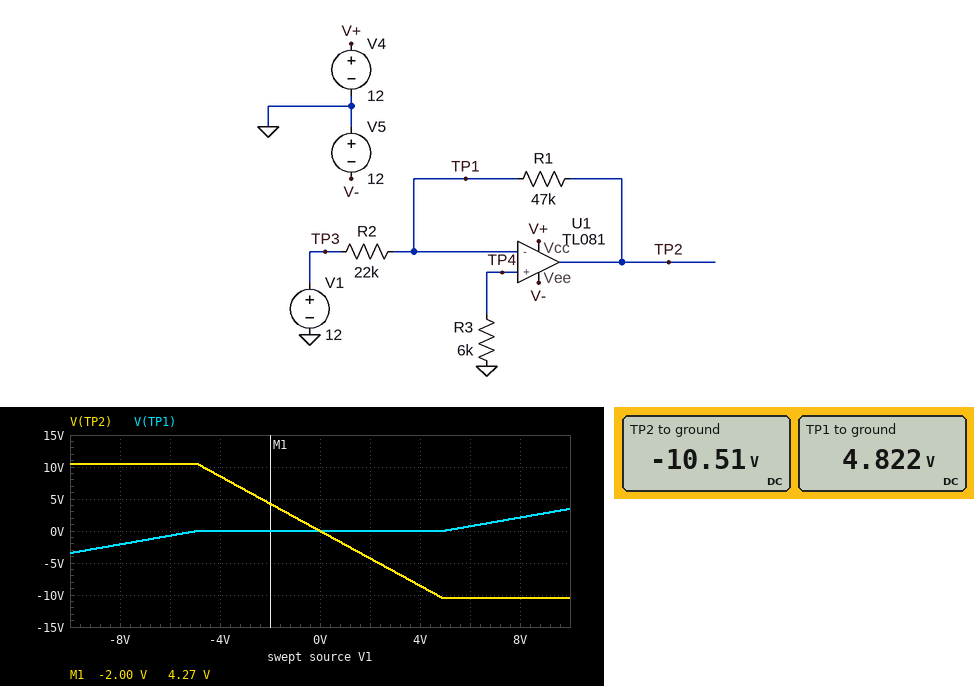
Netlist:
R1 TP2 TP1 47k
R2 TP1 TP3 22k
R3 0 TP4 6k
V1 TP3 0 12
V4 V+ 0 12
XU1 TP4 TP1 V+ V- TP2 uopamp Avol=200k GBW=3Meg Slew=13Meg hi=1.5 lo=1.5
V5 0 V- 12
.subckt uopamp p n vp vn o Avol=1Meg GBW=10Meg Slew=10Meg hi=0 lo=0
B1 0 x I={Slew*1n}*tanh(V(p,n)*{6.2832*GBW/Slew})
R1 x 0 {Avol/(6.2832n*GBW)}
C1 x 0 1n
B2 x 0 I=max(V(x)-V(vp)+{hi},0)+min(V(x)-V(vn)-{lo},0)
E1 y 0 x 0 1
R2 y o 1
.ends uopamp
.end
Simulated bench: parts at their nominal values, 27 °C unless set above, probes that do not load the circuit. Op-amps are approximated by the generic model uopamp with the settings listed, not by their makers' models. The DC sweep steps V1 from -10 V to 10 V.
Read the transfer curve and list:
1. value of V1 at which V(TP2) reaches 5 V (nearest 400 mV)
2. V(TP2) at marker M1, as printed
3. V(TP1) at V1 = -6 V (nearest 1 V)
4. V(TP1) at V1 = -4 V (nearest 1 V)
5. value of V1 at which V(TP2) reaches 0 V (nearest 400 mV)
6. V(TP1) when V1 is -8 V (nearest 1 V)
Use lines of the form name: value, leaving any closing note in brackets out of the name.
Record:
value of V1 at which V(TP2) reaches 5 V: -2.4 V
V(TP2) at marker M1, as printed: 4.27 V
V(TP1) at V1 = -6 V: -1 V
V(TP1) at V1 = -4 V: 0 V
value of V1 at which V(TP2) reaches 0 V: 0 V
V(TP1) when V1 is -8 V: -2 V
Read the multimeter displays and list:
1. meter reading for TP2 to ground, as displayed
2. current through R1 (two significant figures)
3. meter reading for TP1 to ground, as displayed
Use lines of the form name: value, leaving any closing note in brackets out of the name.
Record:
meter reading for TP2 to ground, as displayed: -10.51 V
current through R1: 330 µA
meter reading for TP1 to ground, as displayed: 4.822 V
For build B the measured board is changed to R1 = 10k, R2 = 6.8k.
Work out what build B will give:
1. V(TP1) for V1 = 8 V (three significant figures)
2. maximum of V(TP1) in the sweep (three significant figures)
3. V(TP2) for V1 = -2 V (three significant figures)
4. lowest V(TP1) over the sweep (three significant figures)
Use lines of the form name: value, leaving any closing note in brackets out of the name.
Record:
V(TP1) for V1 = 8 V: 509 mV
maximum of V(TP1) in the sweep: 1.70 V
V(TP2) for V1 = -2 V: 2.94 V
lowest V(TP1) over the sweep: -1.70 V
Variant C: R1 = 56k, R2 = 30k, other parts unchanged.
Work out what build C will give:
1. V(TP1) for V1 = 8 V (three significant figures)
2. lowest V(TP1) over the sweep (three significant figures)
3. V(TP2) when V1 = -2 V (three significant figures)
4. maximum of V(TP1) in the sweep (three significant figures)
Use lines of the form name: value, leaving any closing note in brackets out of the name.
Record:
V(TP1) for V1 = 8 V: 1.54 V
lowest V(TP1) over the sweep: -2.84 V
V(TP2) when V1 = -2 V: 3.73 V
maximum of V(TP1) in the sweep: 2.84 V
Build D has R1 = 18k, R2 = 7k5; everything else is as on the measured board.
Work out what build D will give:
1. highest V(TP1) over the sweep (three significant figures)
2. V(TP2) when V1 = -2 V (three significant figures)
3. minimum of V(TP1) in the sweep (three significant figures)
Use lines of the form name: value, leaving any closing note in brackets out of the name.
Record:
highest V(TP1) over the sweep: 3.97 V
V(TP2) when V1 = -2 V: 4.80 V
minimum of V(TP1) in the sweep: -3.97 V
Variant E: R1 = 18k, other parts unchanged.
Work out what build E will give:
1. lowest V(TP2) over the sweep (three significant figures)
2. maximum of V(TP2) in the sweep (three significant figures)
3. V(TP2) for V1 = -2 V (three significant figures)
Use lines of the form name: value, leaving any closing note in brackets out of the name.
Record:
lowest V(TP2) over the sweep: -8.18 V
maximum of V(TP2) in the sweep: 8.18 V
V(TP2) for V1 = -2 V: 1.64 V
